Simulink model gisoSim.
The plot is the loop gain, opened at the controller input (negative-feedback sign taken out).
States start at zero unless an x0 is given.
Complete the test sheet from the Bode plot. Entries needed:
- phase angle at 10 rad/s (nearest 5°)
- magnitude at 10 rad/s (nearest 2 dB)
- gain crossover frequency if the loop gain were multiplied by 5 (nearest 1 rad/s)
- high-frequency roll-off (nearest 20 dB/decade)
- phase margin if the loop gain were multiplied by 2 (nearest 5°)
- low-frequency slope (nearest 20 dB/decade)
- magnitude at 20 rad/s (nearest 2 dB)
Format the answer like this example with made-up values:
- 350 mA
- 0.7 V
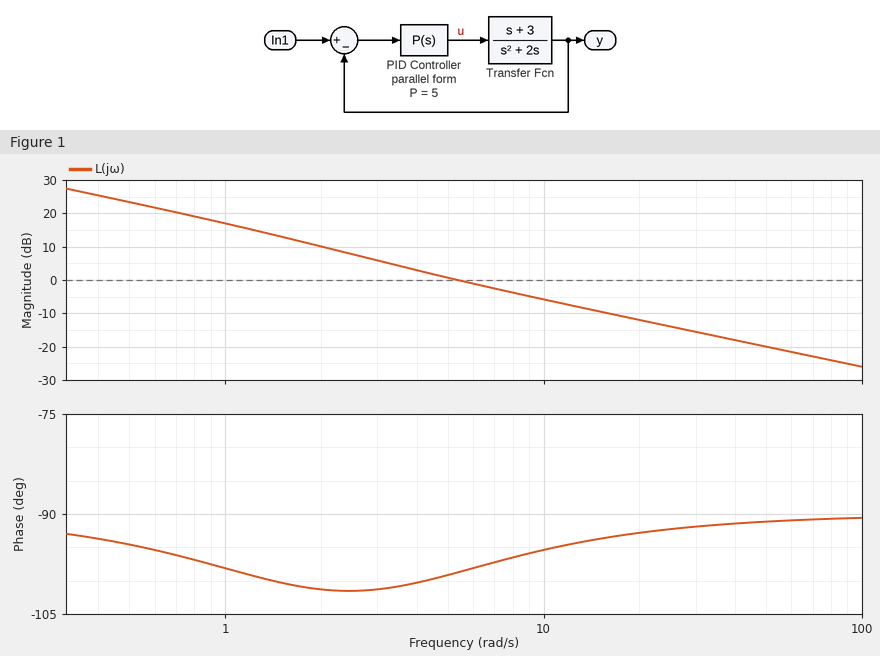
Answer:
- -95°
- -6 dB
- 25 rad/s
- -20 dB/decade
- 85°
- -20 dB/decade
- -12 dB
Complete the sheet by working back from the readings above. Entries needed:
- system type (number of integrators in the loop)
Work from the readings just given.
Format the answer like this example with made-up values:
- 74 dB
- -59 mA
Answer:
- 1
